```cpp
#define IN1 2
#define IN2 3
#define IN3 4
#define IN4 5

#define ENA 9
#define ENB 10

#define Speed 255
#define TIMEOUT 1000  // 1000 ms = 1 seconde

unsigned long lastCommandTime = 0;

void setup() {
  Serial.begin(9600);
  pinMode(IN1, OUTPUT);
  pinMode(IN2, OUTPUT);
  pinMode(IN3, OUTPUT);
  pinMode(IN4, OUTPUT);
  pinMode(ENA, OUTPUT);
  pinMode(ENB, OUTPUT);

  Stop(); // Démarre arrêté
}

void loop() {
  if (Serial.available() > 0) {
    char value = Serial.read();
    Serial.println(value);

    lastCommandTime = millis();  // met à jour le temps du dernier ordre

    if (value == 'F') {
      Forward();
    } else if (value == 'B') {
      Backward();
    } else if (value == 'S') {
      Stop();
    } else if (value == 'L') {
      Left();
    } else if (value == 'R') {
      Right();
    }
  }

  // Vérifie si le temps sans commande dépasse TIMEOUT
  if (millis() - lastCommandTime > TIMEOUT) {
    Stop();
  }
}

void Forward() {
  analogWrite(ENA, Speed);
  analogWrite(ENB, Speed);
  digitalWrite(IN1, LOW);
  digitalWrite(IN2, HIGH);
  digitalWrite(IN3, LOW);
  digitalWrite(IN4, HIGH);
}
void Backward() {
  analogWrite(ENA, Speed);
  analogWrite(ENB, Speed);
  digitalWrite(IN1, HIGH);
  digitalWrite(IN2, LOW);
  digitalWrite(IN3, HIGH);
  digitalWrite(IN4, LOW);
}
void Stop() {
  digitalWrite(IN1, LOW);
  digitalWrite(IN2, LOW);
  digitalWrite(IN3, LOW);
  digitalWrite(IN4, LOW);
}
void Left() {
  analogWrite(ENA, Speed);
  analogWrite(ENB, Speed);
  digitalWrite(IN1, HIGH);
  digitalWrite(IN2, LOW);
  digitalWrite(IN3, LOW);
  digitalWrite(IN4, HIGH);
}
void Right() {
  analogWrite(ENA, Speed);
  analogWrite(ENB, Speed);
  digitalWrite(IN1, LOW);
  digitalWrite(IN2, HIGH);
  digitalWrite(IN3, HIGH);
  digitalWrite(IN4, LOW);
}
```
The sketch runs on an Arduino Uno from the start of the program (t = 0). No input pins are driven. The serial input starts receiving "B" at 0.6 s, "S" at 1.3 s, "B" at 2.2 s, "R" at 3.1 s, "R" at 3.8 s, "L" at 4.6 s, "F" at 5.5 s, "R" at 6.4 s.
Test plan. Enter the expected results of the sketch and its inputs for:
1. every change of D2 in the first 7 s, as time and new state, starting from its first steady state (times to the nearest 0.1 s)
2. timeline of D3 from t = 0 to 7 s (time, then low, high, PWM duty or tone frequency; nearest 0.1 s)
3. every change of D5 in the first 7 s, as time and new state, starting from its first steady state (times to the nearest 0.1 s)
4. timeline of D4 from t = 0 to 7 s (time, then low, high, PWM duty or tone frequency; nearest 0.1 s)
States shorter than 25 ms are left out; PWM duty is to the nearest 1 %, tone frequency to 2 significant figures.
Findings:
0 s low; 0.6 s high; 1.3 s low; 2.2 s high; 3.1 s low; 4.6 s high; 5.5 s low
0 s low; 3.1 s high; 4.6 s low; 5.5 s high
0 s low; 4.6 s high; 6.4 s low
0 s low; 0.6 s high; 1.3 s low; 2.2 s high; 4.6 s low; 6.4 s high
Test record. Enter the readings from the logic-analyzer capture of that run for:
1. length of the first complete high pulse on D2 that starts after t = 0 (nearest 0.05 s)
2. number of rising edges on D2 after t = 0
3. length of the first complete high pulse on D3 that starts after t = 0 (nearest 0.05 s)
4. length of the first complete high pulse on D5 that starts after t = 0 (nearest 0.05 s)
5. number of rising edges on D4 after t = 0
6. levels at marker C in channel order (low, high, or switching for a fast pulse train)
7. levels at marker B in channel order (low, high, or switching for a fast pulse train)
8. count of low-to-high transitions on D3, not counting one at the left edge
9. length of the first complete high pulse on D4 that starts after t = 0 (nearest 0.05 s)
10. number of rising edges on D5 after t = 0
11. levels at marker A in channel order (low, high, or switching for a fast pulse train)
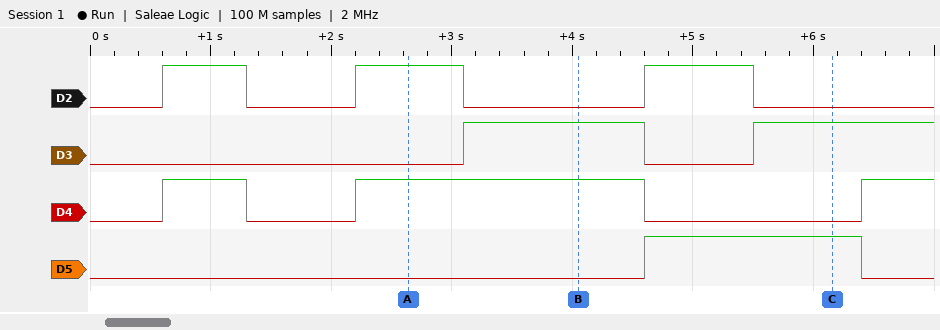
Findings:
0.70 s
3
1.50 s
1.80 s
3
D2 low, D3 high, D4 low, D5 high
D2 low, D3 high, D4 high, D5 low
2
0.70 s
1
D2 high, D3 low, D4 high, D5 low
